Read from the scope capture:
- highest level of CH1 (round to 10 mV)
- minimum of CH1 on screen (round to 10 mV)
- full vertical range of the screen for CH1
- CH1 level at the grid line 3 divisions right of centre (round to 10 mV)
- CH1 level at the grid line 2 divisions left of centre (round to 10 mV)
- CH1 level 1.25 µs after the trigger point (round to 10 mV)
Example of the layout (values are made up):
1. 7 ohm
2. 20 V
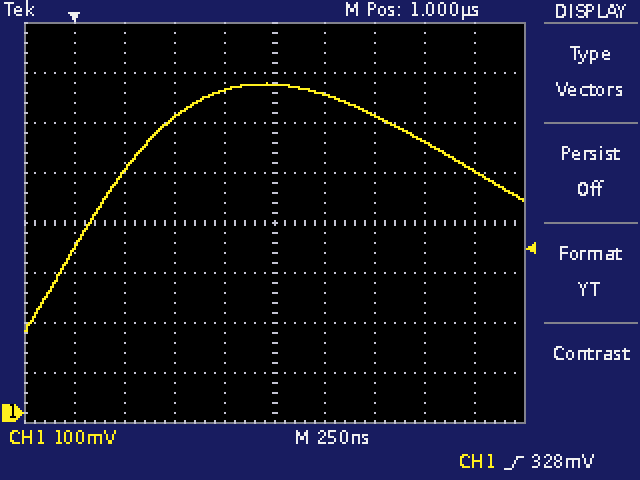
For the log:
1. 660 mV
2. 160 mV
3. 800 mV
4. 540 mV
5. 590 mV
6. 640 mV
